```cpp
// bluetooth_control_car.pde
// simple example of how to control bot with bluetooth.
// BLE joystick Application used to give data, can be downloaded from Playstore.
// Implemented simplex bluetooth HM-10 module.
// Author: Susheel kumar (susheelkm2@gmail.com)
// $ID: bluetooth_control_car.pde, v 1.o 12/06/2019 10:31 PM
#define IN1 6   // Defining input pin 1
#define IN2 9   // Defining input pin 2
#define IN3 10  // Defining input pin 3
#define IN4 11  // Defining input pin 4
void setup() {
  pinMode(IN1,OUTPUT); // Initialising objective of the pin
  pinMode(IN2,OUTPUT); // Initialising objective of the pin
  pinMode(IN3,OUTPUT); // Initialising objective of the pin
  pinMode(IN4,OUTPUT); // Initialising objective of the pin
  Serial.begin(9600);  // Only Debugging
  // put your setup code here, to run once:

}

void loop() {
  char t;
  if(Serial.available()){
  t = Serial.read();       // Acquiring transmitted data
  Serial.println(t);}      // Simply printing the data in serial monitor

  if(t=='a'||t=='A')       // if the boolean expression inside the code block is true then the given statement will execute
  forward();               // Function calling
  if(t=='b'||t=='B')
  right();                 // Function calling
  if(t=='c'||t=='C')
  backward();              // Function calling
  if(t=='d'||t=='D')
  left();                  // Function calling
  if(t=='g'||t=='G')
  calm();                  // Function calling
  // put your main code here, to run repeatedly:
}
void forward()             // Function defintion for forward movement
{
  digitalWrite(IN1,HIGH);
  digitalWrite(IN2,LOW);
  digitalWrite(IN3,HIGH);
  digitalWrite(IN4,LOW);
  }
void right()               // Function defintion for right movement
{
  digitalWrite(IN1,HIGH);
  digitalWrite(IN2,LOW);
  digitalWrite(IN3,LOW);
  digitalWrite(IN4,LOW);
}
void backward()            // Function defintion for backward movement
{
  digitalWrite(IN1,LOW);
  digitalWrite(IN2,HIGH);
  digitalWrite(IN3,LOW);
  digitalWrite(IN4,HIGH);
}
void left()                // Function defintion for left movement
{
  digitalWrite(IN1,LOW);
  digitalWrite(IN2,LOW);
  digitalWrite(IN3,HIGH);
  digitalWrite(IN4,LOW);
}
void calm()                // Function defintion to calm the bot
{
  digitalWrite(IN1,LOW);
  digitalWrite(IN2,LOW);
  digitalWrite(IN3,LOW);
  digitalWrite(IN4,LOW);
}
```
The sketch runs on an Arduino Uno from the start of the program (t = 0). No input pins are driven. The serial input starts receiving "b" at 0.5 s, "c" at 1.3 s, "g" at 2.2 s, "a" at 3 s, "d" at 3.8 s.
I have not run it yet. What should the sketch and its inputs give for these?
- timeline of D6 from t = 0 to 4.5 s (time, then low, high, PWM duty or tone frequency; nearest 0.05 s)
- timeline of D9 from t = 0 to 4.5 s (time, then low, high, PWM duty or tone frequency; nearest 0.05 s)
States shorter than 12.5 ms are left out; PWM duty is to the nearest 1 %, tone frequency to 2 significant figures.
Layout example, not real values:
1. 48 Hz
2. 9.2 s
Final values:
1. 0 s low; 0.5 s high; 1.3 s low; 3 s high; 3.8 s low
2. 0 s low; 1.3 s high; 2.2 s low
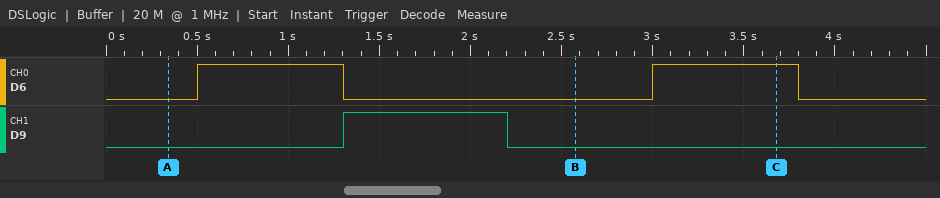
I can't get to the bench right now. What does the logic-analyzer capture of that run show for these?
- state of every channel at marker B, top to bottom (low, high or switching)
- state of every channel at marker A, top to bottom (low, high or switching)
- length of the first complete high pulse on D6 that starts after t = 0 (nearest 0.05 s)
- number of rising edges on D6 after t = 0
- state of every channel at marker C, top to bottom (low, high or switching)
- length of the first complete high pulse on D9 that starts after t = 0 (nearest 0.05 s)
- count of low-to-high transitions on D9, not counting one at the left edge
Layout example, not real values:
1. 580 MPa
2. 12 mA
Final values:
1. D6 low, D9 low
2. D6 low, D9 low
3. 0.80 s
4. 2
5. D6 high, D9 low
6. 0.90 s
7. 1
